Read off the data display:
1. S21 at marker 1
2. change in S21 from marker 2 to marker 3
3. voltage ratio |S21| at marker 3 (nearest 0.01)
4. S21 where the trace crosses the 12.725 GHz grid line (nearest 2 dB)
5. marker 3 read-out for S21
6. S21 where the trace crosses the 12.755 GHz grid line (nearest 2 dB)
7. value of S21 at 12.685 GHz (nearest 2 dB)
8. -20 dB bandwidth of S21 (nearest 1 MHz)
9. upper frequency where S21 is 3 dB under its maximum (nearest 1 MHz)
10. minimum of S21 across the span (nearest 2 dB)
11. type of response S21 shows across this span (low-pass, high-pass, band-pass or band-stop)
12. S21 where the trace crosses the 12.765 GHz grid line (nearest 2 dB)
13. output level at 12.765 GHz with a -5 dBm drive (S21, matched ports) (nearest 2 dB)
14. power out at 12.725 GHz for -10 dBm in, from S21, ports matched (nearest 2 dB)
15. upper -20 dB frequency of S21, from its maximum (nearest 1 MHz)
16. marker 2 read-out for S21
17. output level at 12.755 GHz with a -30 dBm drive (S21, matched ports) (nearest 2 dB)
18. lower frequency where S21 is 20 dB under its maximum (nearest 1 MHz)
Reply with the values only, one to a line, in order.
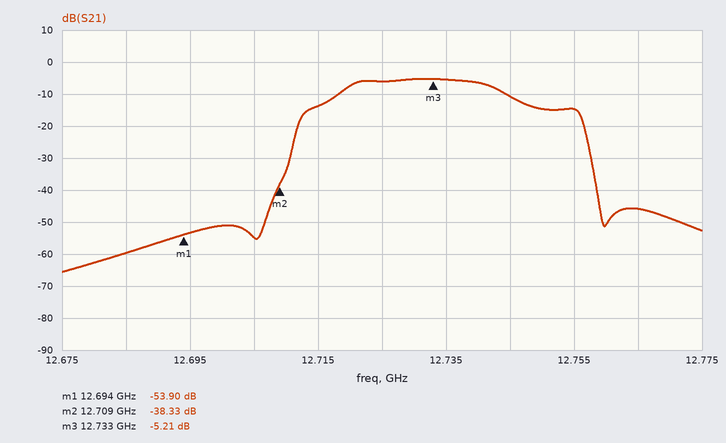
-53.90 dB
33.12 dB
0.55
-6 dB
-5.21 dB
-14 dB
-60 dB
46 MHz
12.743 GHz
-66 dB
band-pass
-46 dB
-50 dBm
-16 dBm
12.757 GHz
-38.33 dB
-44 dBm
12.711 GHz
